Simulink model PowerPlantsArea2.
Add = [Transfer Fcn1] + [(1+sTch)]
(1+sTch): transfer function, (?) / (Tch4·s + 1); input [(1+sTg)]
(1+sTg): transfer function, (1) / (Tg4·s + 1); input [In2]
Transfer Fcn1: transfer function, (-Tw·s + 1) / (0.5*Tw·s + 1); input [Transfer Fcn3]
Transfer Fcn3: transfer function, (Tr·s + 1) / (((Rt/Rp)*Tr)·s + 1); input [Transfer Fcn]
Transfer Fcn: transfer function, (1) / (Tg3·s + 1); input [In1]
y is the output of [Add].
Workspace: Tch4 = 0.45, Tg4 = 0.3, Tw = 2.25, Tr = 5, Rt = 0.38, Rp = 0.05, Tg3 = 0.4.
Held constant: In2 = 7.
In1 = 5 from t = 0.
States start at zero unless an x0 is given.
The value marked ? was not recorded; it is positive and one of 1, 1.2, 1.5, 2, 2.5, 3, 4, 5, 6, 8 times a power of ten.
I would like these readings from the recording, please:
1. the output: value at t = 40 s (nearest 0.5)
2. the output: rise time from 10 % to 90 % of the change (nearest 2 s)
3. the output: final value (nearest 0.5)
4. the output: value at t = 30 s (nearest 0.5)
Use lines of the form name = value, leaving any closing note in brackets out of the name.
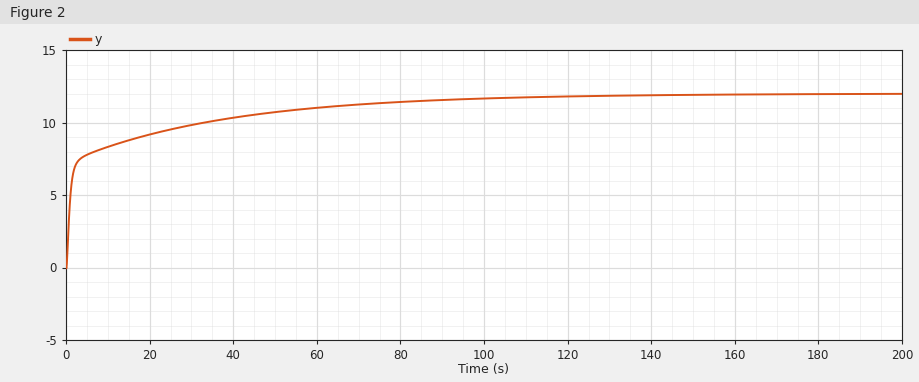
the output: value at t = 40 s = 10.5
the output: rise time from 10 % to 90 % of the change = 52 s
the output: final value = 12.0
the output: value at t = 30 s = 10.0
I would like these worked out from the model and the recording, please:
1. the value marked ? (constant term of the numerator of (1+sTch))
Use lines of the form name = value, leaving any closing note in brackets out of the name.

the value marked ? (constant term of the numerator of (1+sTch)) = 1
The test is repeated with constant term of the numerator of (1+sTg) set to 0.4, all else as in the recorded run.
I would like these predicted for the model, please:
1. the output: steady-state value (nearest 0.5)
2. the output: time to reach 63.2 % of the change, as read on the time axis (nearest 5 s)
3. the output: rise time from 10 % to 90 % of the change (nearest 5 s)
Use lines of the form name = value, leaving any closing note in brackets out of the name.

the output: steady-state value = 8.0
the output: time to reach 63.2 % of the change, as read on the time axis = 20 s
the output: rise time from 10 % to 90 % of the change = 70 s
